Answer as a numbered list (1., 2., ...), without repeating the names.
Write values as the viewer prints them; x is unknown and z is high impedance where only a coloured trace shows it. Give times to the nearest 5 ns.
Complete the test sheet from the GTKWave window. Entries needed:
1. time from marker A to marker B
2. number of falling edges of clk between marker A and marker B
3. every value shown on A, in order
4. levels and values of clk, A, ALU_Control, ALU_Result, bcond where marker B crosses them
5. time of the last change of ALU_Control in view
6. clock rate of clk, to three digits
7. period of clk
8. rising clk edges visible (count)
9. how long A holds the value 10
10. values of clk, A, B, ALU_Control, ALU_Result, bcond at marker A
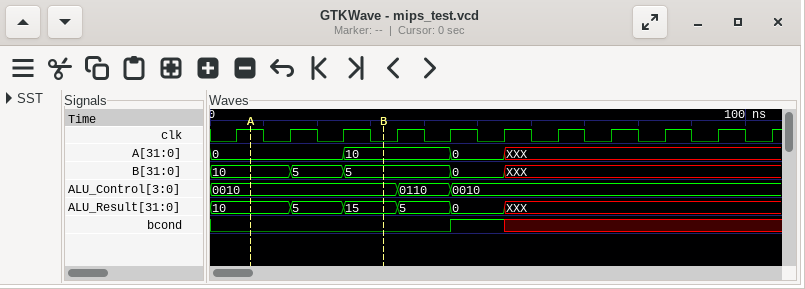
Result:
1. 25 ns
2. 3
3. 0, 10, 0, XXX
4. clk=0, A=10, ALU_Control=0010, ALU_Result=15, bcond=0
5. 45 ns
6. 100 MHz
7. 10 ns
8. 11
9. 20 ns
10. clk=1, A=0, B=10, ALU_Control=0010, ALU_Result=10, bcond=0
